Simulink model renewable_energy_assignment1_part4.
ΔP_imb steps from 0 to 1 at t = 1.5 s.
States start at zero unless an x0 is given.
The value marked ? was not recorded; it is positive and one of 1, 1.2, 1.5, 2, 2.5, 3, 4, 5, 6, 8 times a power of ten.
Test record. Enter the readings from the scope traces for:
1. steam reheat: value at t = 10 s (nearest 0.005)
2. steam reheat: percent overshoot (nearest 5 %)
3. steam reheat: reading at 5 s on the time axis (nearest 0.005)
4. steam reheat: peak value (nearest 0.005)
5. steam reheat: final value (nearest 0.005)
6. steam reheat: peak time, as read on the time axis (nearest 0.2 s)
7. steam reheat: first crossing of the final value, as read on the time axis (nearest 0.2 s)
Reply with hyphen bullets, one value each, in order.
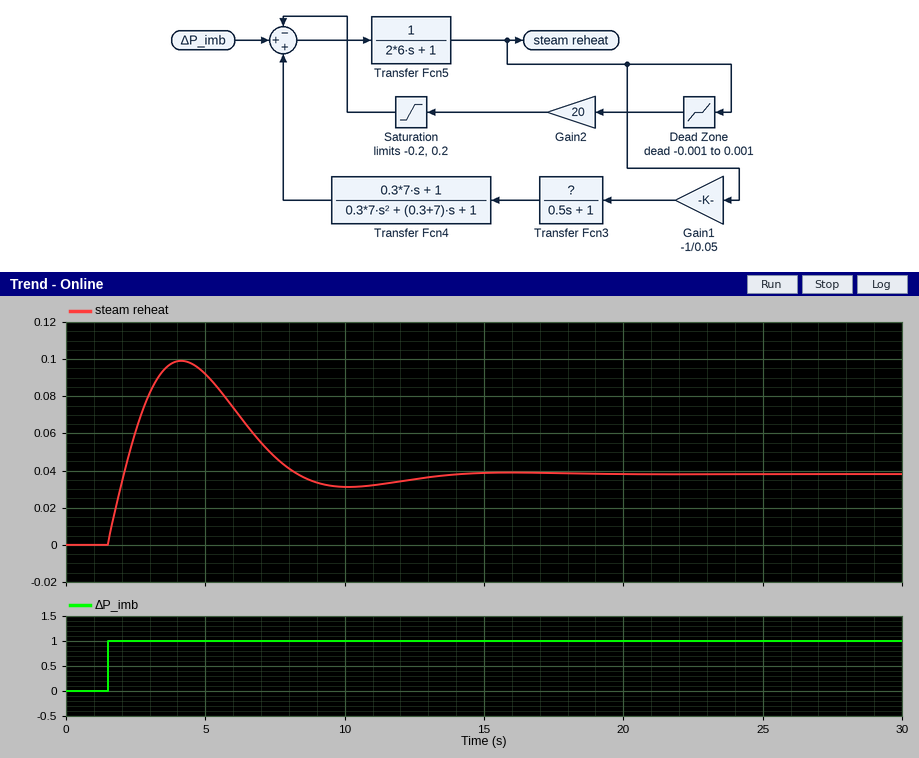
- 0.030
- 160 %
- 0.090
- 0.100
- 0.040
- 4.2 s
- 2.0 s
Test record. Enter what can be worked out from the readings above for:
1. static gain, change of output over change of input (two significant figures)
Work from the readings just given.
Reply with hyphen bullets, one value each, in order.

- 0.040
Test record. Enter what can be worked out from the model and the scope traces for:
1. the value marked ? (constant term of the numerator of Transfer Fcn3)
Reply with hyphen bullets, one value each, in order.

- 1
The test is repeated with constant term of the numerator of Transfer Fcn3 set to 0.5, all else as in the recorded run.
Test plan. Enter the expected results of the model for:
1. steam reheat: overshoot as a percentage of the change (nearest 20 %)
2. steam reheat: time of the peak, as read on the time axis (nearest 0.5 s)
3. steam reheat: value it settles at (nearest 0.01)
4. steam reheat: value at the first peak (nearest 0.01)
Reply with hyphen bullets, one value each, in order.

- 100 %
- 5.5 s
- 0.07
- 0.14
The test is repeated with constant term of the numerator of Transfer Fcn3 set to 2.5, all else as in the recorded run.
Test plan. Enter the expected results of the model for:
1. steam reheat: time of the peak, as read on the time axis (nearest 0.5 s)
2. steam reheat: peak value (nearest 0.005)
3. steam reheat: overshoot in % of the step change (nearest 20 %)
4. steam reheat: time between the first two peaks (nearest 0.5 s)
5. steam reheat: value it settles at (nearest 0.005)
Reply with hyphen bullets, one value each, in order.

- 3.0 s
- 0.065
- 300 %
- 5.0 s
- 0.015
